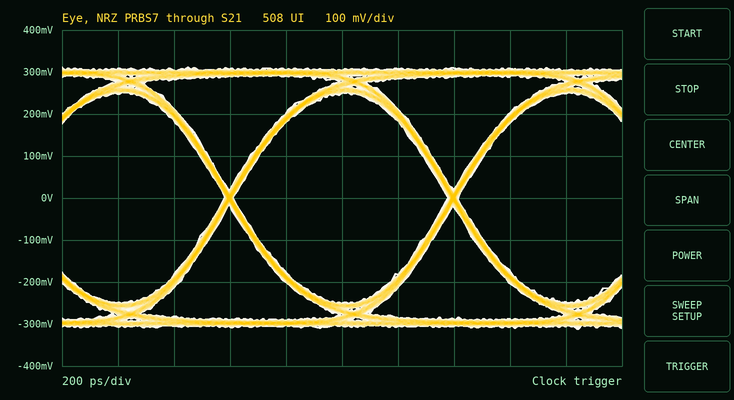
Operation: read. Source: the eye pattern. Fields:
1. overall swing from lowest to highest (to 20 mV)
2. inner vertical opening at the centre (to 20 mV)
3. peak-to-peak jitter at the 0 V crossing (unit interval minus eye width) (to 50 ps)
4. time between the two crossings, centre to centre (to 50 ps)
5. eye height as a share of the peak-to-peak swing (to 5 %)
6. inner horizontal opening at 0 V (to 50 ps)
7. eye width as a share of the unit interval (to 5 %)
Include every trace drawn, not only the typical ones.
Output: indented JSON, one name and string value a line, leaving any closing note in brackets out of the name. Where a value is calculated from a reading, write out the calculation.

{
  "overall swing from lowest to highest": "620 mV",
  "inner vertical opening at the centre": "500 mV",
  "peak-to-peak jitter at the 0 V crossing (unit interval minus eye width)": "50 ps",
  "time between the two crossings, centre to centre": "800 ps",
  "eye height as a share of the peak-to-peak swing": "500 mV / 620 mV ≈ 80.6 %, so 80 % to the nearest 5 %",
  "inner horizontal opening at 0 V": "750 ps",
  "eye width as a share of the unit interval": "750 ps / 800 ps ≈ 93.7 %, so 95 % to the nearest 5 %"
}
